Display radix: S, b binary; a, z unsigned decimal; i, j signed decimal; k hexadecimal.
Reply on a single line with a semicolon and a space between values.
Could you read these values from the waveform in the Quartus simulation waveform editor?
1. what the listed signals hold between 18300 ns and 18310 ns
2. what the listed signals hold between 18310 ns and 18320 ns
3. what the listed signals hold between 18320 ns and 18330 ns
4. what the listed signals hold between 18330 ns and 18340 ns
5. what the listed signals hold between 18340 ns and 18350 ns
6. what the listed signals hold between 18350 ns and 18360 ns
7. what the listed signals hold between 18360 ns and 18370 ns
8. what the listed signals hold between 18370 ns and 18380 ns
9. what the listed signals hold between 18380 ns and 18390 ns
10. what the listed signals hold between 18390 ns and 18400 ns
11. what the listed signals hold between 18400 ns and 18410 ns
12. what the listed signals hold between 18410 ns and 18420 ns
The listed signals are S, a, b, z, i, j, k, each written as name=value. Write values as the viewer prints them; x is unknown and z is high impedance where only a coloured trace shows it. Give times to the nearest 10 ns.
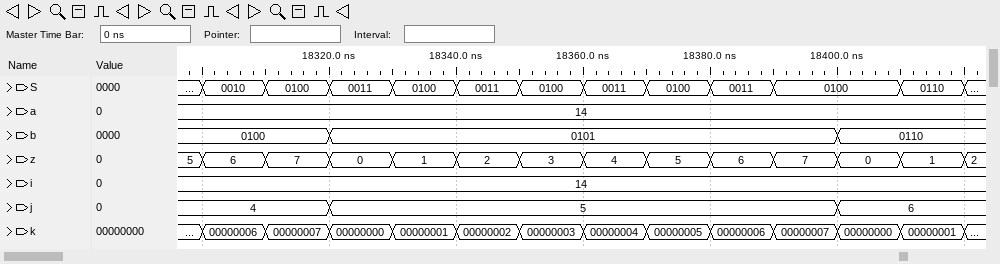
S=0010, a=14, b=0100, z=6, i=14, j=4, k=00000006; S=0100, a=14, b=0100, z=7, i=14, j=4, k=00000007; S=0011, a=14, b=0101, z=0, i=14, j=5, k=00000000; S=0100, a=14, b=0101, z=1, i=14, j=5, k=00000001; S=0011, a=14, b=0101, z=2, i=14, j=5, k=00000002; S=0100, a=14, b=0101, z=3, i=14, j=5, k=00000003; S=0011, a=14, b=0101, z=4, i=14, j=5, k=00000004; S=0100, a=14, b=0101, z=5, i=14, j=5, k=00000005; S=0011, a=14, b=0101, z=6, i=14, j=5, k=00000006; S=0100, a=14, b=0101, z=7, i=14, j=5, k=00000007; S=0100, a=14, b=0110, z=0, i=14, j=6, k=00000000; S=0110, a=14, b=0110, z=1, i=14, j=6, k=00000001
